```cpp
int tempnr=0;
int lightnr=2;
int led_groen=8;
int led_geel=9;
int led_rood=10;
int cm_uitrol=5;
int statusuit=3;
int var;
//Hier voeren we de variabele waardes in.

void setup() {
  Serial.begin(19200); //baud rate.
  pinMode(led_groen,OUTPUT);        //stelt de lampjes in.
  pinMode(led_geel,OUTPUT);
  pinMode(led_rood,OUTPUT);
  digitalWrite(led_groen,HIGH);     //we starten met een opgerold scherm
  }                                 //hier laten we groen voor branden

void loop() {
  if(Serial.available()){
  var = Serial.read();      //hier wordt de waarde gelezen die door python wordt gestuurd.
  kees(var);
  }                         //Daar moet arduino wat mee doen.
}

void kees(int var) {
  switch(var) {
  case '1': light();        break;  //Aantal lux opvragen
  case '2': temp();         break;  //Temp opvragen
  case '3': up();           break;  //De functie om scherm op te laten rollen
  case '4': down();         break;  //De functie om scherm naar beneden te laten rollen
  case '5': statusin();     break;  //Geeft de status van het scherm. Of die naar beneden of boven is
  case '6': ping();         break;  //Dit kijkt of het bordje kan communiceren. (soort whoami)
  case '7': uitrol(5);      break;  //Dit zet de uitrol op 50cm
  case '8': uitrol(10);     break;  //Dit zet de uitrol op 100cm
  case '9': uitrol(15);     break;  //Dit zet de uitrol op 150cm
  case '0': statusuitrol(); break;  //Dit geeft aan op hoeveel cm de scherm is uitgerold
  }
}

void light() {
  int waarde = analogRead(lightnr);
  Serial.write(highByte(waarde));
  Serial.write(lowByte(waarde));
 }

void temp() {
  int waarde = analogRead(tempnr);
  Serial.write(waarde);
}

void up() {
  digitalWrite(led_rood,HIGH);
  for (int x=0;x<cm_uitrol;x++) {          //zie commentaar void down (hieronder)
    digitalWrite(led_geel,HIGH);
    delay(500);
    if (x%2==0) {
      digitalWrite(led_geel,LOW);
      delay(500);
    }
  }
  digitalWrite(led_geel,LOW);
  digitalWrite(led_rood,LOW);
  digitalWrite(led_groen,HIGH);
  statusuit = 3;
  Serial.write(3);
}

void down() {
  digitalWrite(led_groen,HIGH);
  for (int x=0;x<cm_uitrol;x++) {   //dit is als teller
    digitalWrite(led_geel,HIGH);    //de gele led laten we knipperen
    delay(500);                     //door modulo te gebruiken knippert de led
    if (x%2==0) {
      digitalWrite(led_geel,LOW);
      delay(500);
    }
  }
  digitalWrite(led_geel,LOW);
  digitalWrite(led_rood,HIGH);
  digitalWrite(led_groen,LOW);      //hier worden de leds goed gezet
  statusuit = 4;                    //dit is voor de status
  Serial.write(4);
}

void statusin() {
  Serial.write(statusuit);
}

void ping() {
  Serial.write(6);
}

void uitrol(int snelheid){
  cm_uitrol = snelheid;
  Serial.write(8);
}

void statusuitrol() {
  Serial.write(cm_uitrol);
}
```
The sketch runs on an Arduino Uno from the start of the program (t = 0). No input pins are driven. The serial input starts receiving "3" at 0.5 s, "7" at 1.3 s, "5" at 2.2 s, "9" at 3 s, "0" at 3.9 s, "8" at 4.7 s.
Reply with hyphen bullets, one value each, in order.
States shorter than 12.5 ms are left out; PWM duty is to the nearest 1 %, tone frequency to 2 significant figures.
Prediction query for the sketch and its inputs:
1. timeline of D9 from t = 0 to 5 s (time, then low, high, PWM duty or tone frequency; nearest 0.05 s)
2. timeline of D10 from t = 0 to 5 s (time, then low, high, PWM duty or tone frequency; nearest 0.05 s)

- 0 s low; 0.5 s high; 1 s low; 1.5 s high; 2.5 s low; 3 s high; 4 s low
- 0 s low; 0.5 s high; 4.5 s low
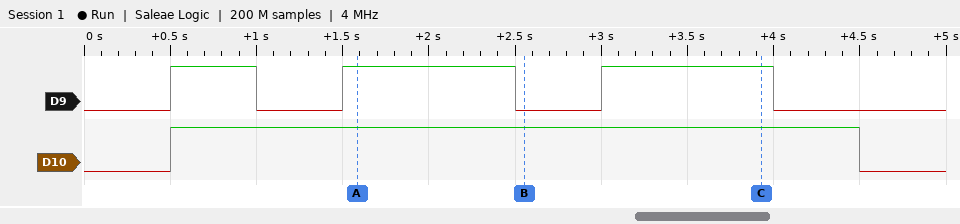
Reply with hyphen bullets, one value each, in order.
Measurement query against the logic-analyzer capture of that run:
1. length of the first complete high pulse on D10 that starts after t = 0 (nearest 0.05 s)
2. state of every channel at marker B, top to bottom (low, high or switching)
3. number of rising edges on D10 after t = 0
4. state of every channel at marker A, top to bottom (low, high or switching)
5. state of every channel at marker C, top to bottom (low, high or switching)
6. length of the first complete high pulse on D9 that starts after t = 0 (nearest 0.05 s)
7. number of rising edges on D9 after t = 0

- 4.00 s
- D9 low, D10 high
- 1
- D9 high, D10 high
- D9 high, D10 high
- 0.50 s
- 3
